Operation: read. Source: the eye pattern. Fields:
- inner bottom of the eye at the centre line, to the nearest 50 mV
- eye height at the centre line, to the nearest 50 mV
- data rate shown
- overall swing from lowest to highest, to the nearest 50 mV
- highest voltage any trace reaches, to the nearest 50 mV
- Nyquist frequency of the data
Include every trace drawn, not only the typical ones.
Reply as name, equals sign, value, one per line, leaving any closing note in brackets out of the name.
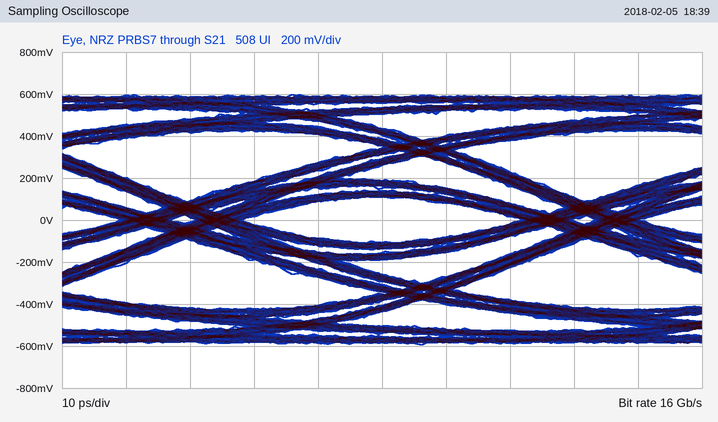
inner bottom of the eye at the centre line, to the nearest 50 mV = -100 mV
eye height at the centre line, to the nearest 50 mV = 200 mV
data rate shown = 16 Gb/s
overall swing from lowest to highest, to the nearest 50 mV = 1.20 V
highest voltage any trace reaches, to the nearest 50 mV = 600 mV
Nyquist frequency of the data = 8 GHz
